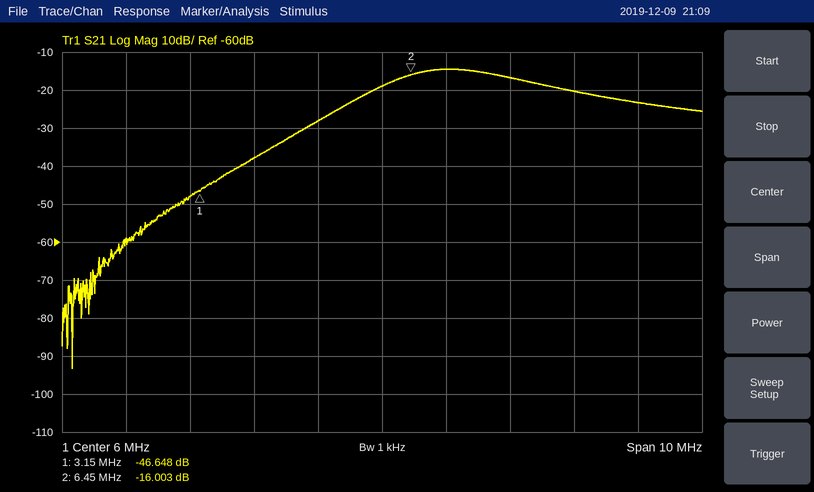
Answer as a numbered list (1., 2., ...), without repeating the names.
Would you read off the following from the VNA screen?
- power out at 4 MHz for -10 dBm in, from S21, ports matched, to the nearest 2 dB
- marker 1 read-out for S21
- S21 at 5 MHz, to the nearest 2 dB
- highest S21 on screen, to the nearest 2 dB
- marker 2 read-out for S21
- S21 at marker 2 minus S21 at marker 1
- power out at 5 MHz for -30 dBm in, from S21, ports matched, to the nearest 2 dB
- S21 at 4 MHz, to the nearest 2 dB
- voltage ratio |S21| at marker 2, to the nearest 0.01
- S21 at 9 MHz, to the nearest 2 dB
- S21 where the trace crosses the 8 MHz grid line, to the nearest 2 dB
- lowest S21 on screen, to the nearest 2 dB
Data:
1. -48 dBm
2. -46.648 dB
3. -28 dB
4. -14 dB
5. -16.003 dB
6. 30.645 dB
7. -58 dBm
8. -38 dB
9. 0.16
10. -20 dB
11. -16 dB
12. -94 dB
